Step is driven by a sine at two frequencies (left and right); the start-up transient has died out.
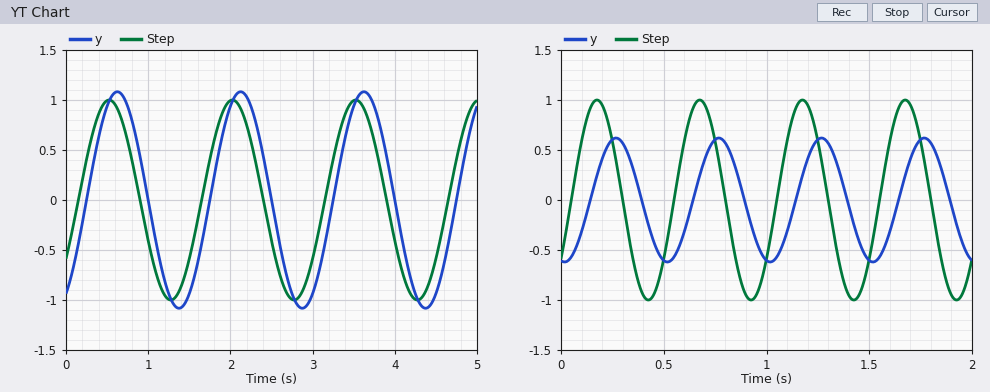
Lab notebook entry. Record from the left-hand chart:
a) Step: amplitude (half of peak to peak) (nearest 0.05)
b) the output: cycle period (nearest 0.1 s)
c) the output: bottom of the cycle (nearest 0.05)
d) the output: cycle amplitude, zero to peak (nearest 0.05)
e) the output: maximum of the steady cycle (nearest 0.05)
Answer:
1.00
1.5 s
-1.10
1.10
1.10
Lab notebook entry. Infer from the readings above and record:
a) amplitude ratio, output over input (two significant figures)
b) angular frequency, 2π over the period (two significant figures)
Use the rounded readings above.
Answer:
1.1
4.2 rad/s
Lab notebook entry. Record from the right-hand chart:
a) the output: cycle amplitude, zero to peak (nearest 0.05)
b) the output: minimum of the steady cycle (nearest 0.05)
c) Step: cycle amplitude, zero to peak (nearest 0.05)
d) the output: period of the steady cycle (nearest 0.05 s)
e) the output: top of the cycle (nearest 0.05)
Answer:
0.60
-0.60
1.00
0.50 s
0.60
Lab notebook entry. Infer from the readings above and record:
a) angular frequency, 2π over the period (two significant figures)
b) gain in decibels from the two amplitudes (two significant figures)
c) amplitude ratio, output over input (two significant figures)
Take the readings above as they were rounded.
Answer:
13 rad/s
-4.4 dB
0.60
